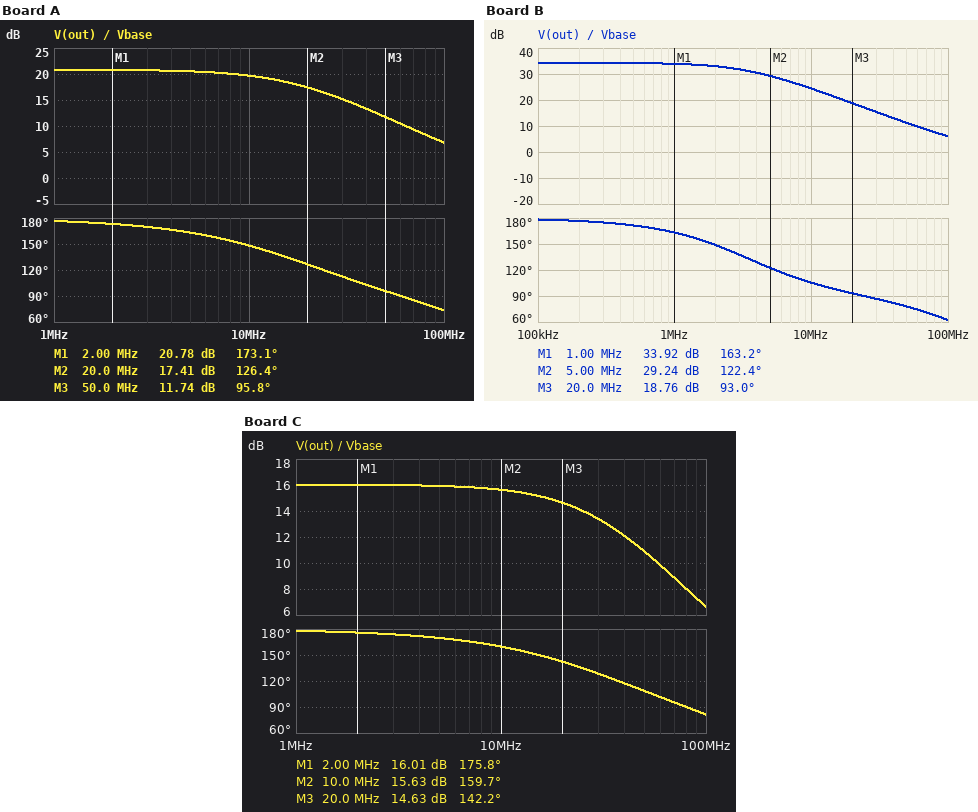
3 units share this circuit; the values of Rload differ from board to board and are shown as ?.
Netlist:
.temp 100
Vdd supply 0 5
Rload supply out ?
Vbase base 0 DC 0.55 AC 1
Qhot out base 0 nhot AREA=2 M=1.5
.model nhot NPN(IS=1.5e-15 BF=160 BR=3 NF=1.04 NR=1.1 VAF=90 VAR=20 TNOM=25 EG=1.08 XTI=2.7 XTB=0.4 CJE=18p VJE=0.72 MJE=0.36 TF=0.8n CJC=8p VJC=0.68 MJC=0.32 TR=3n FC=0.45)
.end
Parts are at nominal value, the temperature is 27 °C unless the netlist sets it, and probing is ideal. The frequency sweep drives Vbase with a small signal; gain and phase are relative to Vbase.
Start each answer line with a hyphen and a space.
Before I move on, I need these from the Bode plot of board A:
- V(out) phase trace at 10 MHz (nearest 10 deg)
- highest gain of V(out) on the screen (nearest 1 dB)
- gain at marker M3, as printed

- 150 deg
- 21 dB
- 11.74 dB
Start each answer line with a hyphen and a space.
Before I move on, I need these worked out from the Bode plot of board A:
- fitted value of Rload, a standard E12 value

- 680 Ω
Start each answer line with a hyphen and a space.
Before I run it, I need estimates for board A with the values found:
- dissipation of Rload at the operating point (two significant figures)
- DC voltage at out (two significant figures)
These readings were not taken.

- 200 µW
- 4.6 V
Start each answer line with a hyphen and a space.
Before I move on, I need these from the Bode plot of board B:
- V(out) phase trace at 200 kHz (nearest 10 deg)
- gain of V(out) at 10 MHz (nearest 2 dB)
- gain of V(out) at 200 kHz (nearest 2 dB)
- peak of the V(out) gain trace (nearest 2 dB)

- 180 deg
- 24 dB
- 34 dB
- 34 dB
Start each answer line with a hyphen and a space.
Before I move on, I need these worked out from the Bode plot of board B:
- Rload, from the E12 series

- 3.3 kΩ
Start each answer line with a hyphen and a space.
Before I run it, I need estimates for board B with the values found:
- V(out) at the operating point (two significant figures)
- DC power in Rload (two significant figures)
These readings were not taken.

- 3.2 V
- 950 µW
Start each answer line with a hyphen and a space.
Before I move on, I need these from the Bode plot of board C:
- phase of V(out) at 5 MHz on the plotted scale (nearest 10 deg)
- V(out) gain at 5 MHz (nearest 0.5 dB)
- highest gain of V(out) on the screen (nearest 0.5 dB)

- 170 deg
- 16.0 dB
- 16.0 dB
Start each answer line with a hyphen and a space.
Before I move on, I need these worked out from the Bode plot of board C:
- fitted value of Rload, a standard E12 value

- 390 Ω
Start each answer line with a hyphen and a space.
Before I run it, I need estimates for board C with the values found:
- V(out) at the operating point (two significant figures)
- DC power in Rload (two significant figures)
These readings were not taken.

- 4.8 V
- 120 µW
